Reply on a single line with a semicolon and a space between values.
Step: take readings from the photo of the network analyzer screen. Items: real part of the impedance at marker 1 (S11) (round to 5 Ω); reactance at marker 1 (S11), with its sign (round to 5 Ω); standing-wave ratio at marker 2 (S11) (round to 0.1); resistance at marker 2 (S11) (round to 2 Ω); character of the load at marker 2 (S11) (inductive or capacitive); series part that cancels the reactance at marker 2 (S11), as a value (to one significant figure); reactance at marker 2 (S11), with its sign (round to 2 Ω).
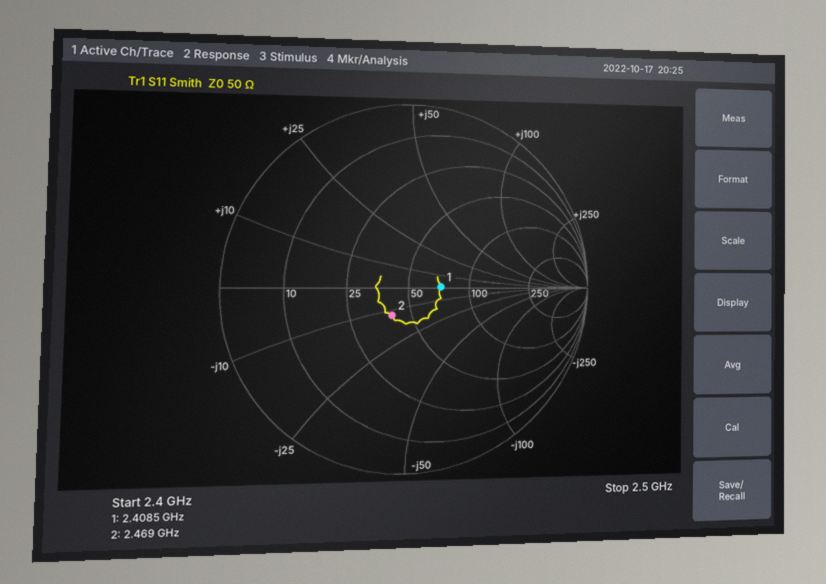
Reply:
70 Ω; 0 Ω; 1.4; 40 Ω; capacitive; 800 pH; -12 Ω
